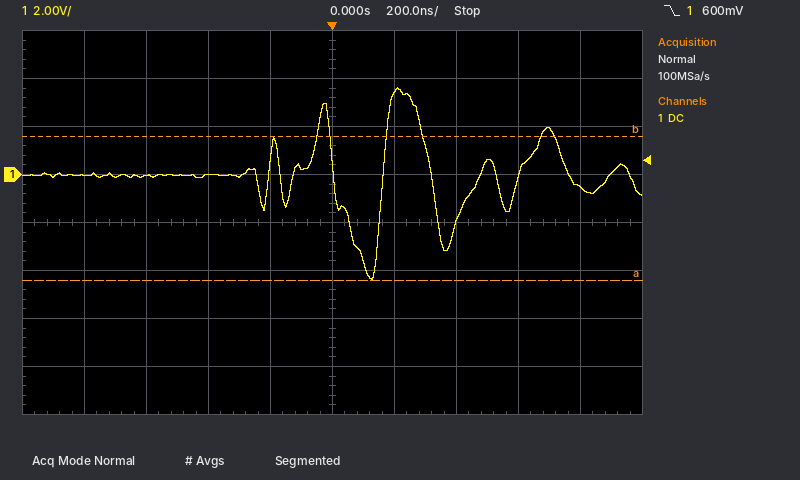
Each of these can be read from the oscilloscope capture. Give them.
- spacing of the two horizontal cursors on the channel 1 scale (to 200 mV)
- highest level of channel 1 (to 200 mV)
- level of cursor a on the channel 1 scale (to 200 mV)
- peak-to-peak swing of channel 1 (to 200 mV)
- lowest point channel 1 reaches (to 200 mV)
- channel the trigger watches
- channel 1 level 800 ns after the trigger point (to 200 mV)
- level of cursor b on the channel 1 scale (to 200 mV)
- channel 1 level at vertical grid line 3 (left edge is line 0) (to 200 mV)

6.0 V
3.6 V
-4.4 V
8.0 V
-4.4 V
channel 1
-600 mV
1.6 V
0.0 V
